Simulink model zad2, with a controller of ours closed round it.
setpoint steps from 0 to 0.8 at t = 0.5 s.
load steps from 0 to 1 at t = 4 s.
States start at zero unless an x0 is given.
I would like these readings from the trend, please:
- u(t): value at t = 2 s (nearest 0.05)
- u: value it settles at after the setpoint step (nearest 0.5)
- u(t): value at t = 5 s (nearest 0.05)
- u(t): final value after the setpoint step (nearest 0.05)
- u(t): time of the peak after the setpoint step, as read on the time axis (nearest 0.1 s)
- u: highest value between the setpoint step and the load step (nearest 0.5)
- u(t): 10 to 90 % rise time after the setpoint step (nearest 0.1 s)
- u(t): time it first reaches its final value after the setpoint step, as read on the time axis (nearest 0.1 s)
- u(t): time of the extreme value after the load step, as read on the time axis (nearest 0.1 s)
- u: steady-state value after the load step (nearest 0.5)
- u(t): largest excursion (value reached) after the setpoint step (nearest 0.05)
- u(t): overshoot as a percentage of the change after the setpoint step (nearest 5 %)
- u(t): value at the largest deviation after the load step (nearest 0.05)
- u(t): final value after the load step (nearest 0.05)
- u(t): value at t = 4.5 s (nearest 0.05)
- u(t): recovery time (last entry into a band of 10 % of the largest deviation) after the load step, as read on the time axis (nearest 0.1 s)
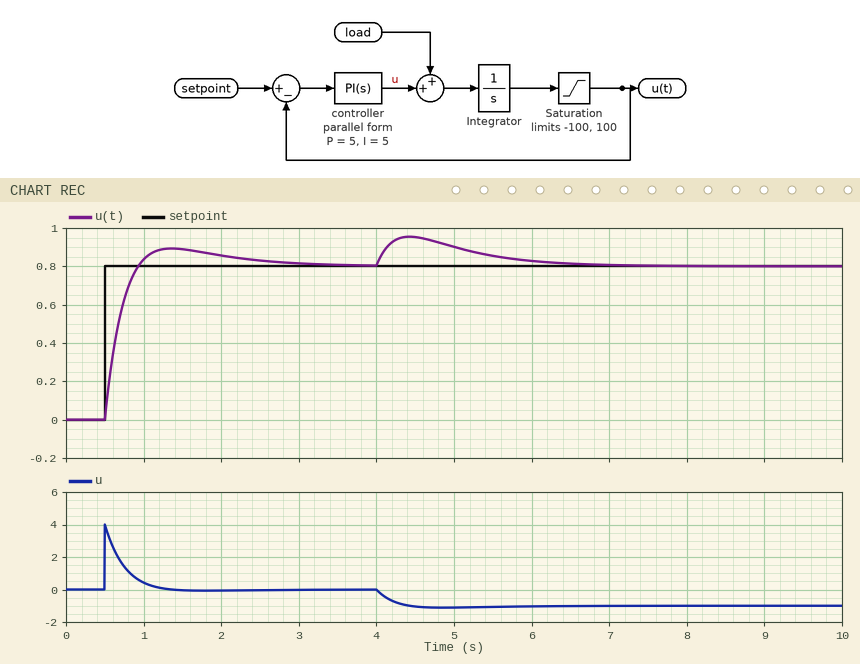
0.85
0.0
0.90
0.80
1.4 s
4.0
0.3 s
0.9 s
4.4 s
-1.0
0.90
10 %
0.95
0.80
0.95
6.5 s
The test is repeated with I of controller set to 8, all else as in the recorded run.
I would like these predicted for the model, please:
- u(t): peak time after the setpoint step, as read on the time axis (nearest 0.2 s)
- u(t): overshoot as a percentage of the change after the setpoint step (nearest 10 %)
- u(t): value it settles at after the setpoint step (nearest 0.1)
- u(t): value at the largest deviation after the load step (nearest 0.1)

1.2 s
20 %
0.8
0.9
